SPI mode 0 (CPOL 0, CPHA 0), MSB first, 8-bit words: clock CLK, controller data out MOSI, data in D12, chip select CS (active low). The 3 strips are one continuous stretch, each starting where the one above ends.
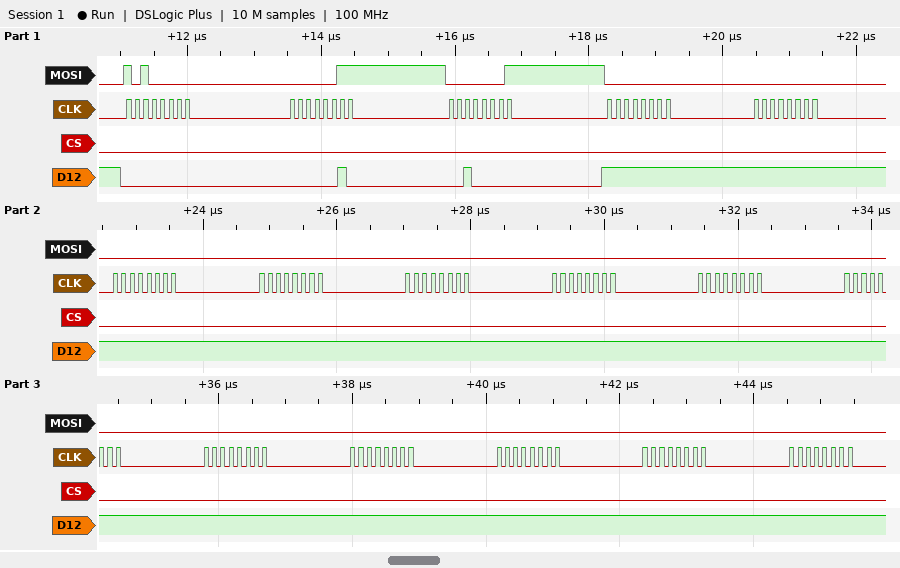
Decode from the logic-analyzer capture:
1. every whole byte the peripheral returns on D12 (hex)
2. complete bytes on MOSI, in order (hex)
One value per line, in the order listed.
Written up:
00 02 20 FF FF FF FF FF FF FF FF FF FF FF FF FF
A0 03 01 00 00 00 00 00 00 00 00 00 00 00 00 00
